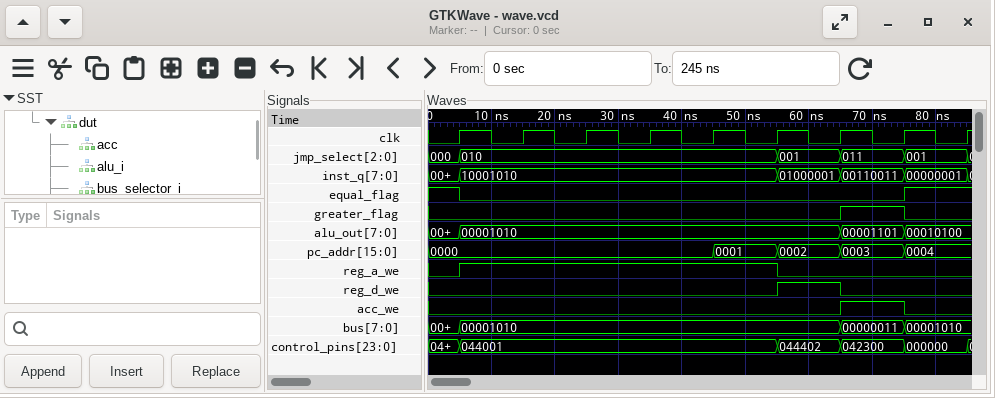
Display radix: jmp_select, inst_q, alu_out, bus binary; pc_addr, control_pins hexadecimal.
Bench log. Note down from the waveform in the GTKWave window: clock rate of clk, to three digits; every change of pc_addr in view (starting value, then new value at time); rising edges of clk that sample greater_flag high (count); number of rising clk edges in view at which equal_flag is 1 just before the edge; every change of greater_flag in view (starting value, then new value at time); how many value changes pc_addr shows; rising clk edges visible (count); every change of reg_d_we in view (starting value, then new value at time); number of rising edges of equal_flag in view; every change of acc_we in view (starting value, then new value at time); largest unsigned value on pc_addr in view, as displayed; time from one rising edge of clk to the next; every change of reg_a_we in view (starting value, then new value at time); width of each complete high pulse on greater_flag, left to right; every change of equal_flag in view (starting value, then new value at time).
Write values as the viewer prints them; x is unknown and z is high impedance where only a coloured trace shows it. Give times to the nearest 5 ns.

100 MHz
0000, 0001 at 45 ns, 0002 at 55 ns, 0003 at 65 ns, 0004 at 75 ns
1
2
0, 1 at 65 ns, 0 at 75 ns
4
9
0, 1 at 55 ns, 0 at 65 ns
1
0, 1 at 65 ns, 0 at 75 ns
0004
10 ns
0, 1 at 5 ns, 0 at 55 ns
10 ns
1, 0 at 5 ns, 1 at 75 ns
